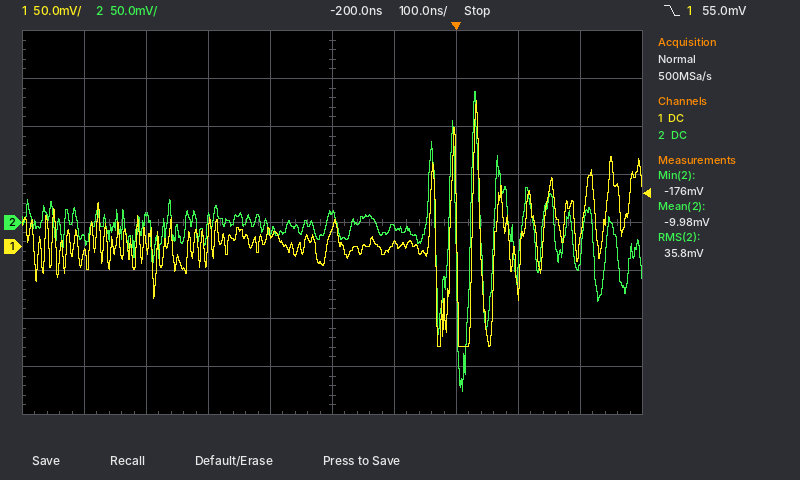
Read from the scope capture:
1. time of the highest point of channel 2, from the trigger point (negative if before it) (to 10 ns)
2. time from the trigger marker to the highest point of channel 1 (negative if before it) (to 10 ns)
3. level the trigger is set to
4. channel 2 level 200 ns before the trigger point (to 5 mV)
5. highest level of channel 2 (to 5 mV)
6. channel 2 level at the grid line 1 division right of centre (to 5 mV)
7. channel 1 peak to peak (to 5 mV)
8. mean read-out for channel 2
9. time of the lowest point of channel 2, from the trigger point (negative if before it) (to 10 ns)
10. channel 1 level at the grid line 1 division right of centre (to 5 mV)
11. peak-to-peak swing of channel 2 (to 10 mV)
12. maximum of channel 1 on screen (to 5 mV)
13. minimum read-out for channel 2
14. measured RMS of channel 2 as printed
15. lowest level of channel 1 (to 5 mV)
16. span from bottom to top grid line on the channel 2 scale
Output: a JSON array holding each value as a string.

["+30 ns", "+30 ns", "55.0 mV", "10 mV", "135 mV", "-5 mV", "255 mV", "-9.98 mV", "+10 ns", "5 mV", "310 mV", "150 mV", "-176 mV", "35.8 mV", "-105 mV", "400 mV"]
